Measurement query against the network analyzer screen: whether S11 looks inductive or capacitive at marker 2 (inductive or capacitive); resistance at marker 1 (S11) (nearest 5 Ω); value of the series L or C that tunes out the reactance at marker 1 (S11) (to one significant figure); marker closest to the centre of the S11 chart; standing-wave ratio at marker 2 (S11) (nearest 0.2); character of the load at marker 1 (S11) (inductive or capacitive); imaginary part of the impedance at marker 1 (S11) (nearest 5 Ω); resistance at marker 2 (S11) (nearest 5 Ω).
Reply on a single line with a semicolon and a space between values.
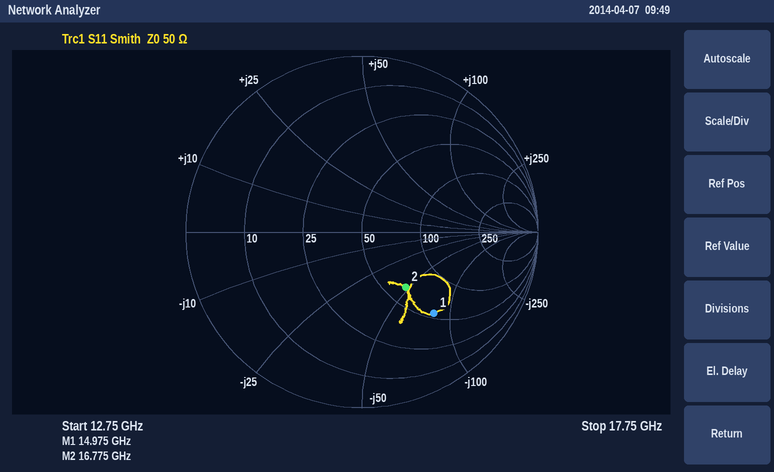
capacitive; 55 Ω; 900 pH; marker 2; 2.4; capacitive; -80 Ω; 65 Ω
